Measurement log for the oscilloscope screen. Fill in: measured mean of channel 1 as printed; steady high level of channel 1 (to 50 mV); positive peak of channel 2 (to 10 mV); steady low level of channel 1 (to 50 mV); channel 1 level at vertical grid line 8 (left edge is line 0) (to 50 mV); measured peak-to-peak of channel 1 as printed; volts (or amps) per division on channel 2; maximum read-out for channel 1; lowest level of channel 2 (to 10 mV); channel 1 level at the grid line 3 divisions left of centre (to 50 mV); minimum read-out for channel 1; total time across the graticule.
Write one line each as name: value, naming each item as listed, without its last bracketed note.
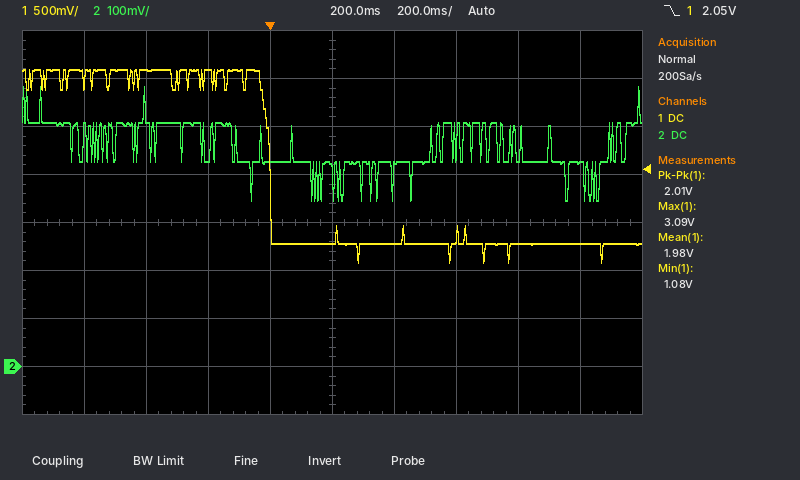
measured mean of channel 1 as printed: 1.98 V
steady high level of channel 1: 3.10 V
positive peak of channel 2: 580 mV
steady low level of channel 1: 1.30 V
channel 1 level at vertical grid line 8 (left edge is line 0): 1.30 V
measured peak-to-peak of channel 1 as printed: 2.01 V
volts (or amps) per division on channel 2: 100 mV
maximum read-out for channel 1: 3.09 V
lowest level of channel 2: 350 mV
channel 1 level at the grid line 3 divisions left of centre: 3.10 V
minimum read-out for channel 1: 1.08 V
total time across the graticule: 2 s
